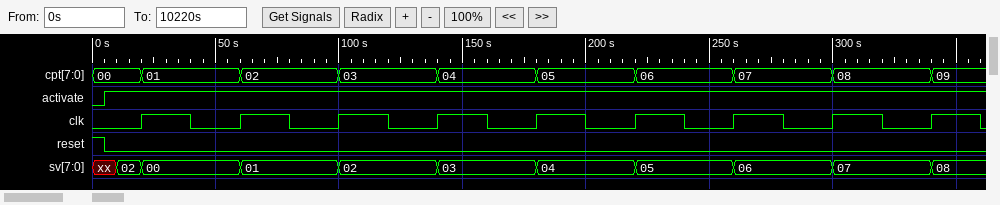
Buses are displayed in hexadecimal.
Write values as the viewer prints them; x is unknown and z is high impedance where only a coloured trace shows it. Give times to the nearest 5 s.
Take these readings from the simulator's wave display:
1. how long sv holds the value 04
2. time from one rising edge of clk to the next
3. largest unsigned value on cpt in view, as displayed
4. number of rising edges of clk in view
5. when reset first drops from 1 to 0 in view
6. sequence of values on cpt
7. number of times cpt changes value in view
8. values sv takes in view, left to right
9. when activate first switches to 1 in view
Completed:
40 s
40 s
09
9
5 s
00, 01, 02, 03, 04, 05, 06, 07, 08, 09
9
xx, 02, 00, 01, 02, 03, 04, 05, 06, 07, 08
5 s
